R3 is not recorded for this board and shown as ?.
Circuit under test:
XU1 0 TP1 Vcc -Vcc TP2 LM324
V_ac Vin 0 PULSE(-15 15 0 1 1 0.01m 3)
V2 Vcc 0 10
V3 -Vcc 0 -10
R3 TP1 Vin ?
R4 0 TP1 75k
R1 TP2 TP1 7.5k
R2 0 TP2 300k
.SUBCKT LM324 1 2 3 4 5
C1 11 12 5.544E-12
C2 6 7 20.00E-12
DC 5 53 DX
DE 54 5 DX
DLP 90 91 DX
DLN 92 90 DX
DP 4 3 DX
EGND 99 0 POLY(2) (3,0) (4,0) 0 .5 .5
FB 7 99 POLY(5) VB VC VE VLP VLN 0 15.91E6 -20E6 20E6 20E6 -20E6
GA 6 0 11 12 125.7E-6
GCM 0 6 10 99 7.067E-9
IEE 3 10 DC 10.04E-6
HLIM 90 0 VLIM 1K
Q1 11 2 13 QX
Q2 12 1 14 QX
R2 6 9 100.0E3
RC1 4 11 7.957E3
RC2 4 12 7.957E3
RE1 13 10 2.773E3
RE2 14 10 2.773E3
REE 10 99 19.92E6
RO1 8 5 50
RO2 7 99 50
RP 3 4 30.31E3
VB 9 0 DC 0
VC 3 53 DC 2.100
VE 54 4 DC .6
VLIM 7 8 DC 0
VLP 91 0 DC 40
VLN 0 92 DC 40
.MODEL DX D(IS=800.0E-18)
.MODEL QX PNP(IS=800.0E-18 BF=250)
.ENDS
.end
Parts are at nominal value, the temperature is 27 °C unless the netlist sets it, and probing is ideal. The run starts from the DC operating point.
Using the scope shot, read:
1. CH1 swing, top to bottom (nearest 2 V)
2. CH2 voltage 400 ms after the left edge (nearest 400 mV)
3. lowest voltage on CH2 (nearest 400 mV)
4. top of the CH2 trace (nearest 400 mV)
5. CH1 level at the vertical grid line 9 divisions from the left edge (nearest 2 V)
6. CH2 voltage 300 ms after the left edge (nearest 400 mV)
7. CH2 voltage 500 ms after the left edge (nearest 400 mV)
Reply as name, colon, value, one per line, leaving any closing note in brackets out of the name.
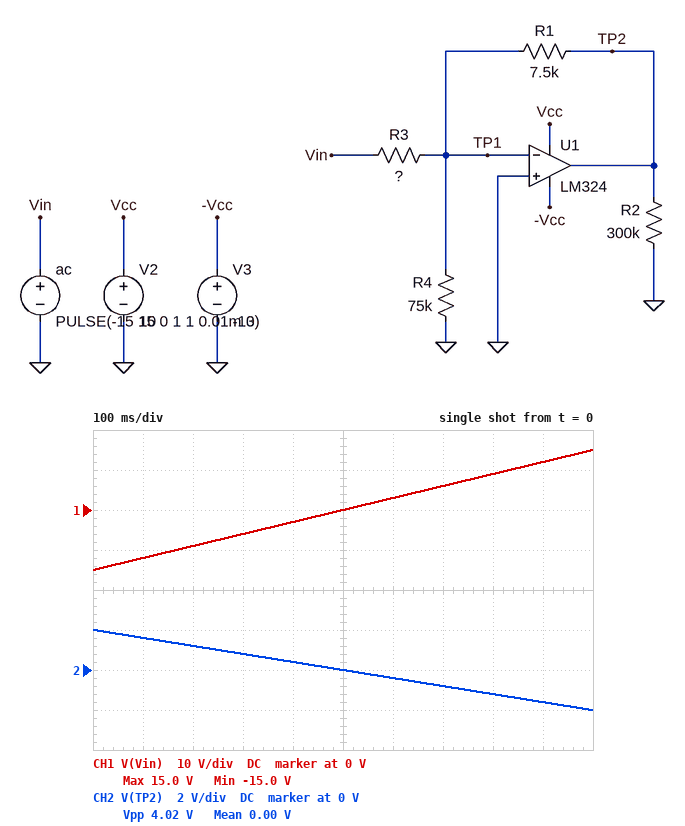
CH1 swing, top to bottom: 30 V
CH2 voltage 400 ms after the left edge: 400 mV
lowest voltage on CH2: -2.0 V
top of the CH2 trace: 2.0 V
CH1 level at the vertical grid line 9 divisions from the left edge: 12 V
CH2 voltage 300 ms after the left edge: 800 mV
CH2 voltage 500 ms after the left edge: 0 V
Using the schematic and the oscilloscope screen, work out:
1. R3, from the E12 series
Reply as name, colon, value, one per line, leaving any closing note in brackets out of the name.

R3, from the E12 series: 56 kΩ
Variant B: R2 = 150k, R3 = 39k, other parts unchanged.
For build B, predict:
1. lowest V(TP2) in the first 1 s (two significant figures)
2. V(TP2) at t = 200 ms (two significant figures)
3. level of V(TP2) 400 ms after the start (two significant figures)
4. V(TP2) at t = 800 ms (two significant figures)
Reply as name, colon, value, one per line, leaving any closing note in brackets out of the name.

lowest V(TP2) in the first 1 s: -2.9 V
V(TP2) at t = 200 ms: 1.7 V
level of V(TP2) 400 ms after the start: 580 mV
V(TP2) at t = 800 ms: -1.7 V
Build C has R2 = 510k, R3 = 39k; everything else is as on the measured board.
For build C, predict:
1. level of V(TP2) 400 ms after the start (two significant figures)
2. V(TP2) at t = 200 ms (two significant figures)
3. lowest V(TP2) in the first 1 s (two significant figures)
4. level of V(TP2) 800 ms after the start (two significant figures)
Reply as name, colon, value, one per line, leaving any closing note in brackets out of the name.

level of V(TP2) 400 ms after the start: 580 mV
V(TP2) at t = 200 ms: 1.7 V
lowest V(TP2) in the first 1 s: -2.9 V
level of V(TP2) 800 ms after the start: -1.7 V
